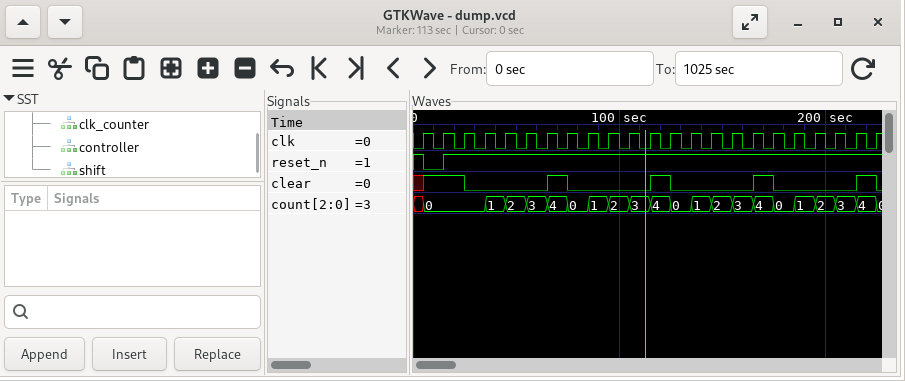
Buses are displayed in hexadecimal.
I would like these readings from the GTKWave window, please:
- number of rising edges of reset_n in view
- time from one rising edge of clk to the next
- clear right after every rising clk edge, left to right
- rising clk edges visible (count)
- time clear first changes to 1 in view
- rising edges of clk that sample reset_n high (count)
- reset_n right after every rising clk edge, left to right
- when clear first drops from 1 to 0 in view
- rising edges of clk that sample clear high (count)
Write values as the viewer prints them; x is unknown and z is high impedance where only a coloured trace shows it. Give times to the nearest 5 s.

1
10 s
1 1 0 0 0 0 1 0 0 0 0 1 0 0 0 0 1 0 0 0 0 1 0
23
5 s
22
0 1 1 1 1 1 1 1 1 1 1 1 1 1 1 1 1 1 1 1 1 1 1
25 s
6
